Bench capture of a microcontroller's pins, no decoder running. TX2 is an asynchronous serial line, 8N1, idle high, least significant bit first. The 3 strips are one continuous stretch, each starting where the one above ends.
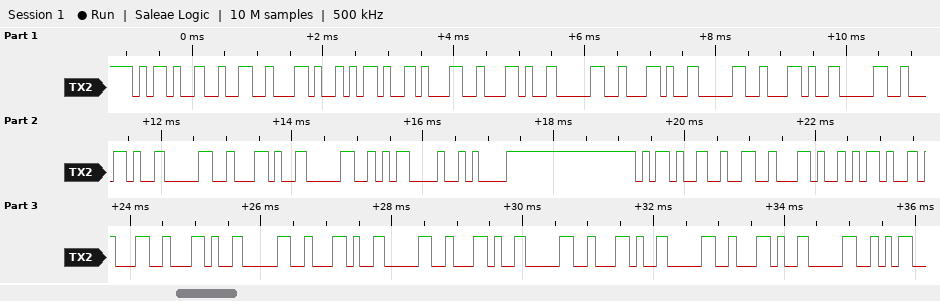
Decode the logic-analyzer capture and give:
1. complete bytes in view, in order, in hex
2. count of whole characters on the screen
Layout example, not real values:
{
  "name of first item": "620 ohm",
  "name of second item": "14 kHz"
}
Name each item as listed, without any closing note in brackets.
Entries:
{
  "complete bytes in view, in order, in hex": "2D 32 2C 2D 31 2C 30 2C 30 2C 30 2C 30 2C 30 0D 0A 2D 32 2C 2D 31 2C 30 2C 30 2C 30 2C 30 2C 30",
  "count of whole characters on the screen": "32"
}
